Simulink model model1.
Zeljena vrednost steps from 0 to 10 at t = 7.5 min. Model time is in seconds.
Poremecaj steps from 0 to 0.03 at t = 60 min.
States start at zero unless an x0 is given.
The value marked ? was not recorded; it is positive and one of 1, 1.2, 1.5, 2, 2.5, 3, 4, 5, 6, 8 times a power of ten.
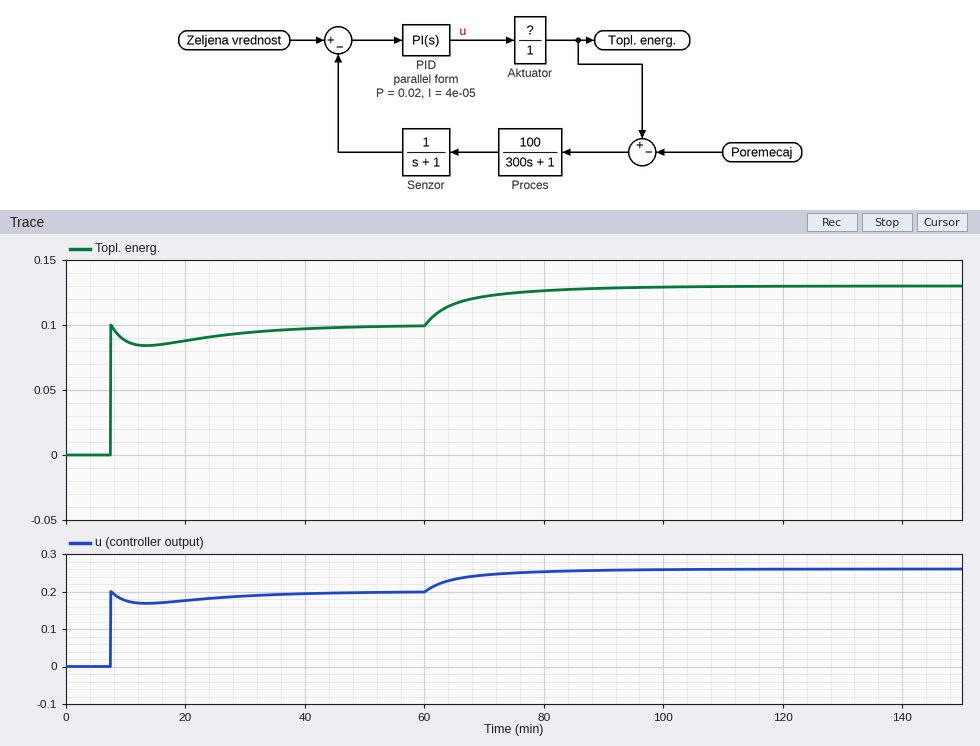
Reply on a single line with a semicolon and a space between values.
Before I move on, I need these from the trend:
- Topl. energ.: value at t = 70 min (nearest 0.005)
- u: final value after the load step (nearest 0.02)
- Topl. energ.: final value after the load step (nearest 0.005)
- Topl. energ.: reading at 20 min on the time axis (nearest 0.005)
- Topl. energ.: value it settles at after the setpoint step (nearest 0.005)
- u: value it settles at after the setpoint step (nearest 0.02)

0.120; 0.26; 0.130; 0.090; 0.100; 0.20
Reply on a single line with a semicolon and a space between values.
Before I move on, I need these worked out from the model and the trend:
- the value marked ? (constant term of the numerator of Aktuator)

0.5
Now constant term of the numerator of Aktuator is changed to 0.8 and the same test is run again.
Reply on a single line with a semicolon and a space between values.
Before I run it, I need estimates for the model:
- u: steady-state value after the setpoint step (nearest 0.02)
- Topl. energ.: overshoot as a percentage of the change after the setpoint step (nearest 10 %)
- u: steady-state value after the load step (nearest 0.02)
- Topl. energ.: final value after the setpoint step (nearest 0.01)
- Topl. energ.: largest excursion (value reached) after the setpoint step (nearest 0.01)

0.12; 60 %; 0.16; 0.10; 0.16
